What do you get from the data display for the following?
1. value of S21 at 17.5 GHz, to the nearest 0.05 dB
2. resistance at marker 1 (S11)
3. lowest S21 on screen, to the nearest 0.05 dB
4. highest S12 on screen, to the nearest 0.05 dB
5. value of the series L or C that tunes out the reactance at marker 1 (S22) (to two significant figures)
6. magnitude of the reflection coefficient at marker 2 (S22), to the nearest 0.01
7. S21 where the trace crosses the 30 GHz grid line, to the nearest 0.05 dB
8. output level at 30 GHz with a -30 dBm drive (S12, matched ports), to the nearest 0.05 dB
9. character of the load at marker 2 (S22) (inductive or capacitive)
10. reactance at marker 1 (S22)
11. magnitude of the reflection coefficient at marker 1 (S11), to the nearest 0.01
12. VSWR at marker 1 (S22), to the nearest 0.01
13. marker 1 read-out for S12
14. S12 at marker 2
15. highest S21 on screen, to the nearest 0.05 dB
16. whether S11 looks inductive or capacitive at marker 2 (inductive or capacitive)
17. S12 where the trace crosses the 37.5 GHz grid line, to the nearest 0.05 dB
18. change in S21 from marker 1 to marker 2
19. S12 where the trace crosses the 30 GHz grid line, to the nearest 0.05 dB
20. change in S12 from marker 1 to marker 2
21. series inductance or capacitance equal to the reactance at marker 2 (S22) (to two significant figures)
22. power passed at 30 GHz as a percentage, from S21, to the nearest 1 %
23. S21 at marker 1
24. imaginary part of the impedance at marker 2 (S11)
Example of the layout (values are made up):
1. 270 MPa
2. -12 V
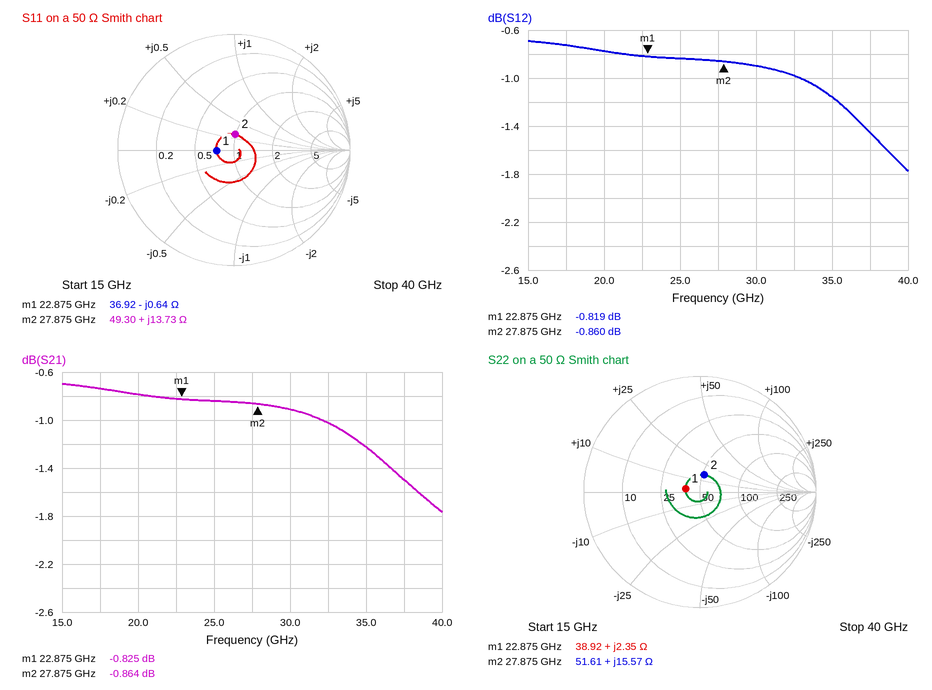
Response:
1. -0.75 dB
2. 36.92 Ω
3. -1.75 dB
4. -0.70 dB
5. 3.0 pF
6. 0.15
7. -0.90 dB
8. -30.90 dBm
9. inductive
10. +2.35 Ω
11. 0.15
12. 1.29
13. -0.819 dB
14. -0.860 dB
15. -0.70 dB
16. inductive
17. -1.45 dB
18. -0.039 dB
19. -0.90 dB
20. -0.041 dB
21. 89 pH
22. 81 %
23. -0.825 dB
24. +13.73 Ω
